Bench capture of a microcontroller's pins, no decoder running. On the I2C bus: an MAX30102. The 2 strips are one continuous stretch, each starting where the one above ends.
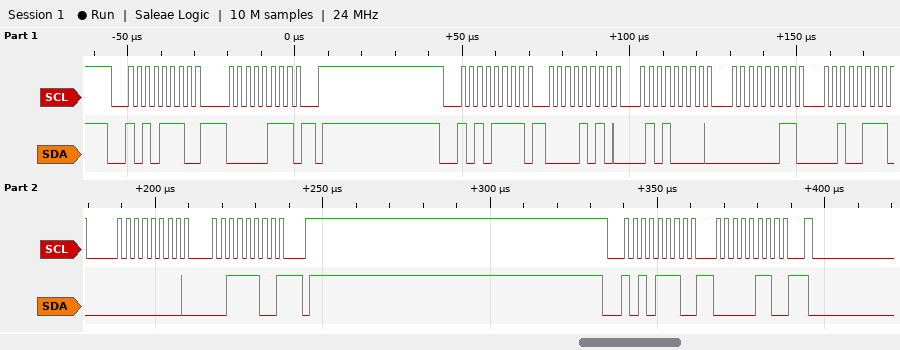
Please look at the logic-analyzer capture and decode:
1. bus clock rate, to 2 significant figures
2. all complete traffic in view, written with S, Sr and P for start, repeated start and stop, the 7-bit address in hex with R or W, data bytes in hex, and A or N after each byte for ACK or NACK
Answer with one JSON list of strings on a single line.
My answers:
["400 kHz", "S 57W A 07 A P S 57R A 0A A 50 A 03 A 27 A 00 A 3C N P S 57W A 06 A"]
